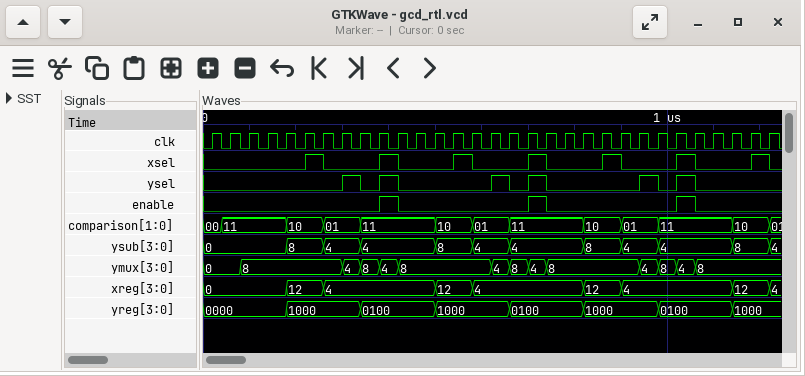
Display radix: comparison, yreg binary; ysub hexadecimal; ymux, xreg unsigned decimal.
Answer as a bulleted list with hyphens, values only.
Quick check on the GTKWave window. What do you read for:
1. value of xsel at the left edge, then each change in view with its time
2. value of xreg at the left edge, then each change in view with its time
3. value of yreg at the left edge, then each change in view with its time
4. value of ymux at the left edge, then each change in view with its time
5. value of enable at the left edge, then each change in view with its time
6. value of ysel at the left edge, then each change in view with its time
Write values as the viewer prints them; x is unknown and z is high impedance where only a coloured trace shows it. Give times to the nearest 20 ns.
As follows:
- 0, 1 at 220 ns, 0 at 260 ns, 1 at 380 ns, 0 at 420 ns, 1 at 540 ns, 0 at 580 ns, 1 at 700 ns, 0 at 740 ns, 1 at 860 ns, 0 at 900 ns, 1 at 1020 ns, 0 at 1060 ns, 1 at 1180 ns, 0 at 1220 ns
- 0, 12 at 180 ns, 4 at 260 ns, 12 at 500 ns, 4 at 580 ns, 12 at 820 ns, 4 at 900 ns, 12 at 1140 ns, 4 at 1220 ns
- 0000, 1000 at 180 ns, 0100 at 340 ns, 1000 at 500 ns, 0100 at 660 ns, 1000 at 820 ns, 0100 at 980 ns, 1000 at 1140 ns
- 0, 8 at 80 ns, 4 at 300 ns, 8 at 340 ns, 4 at 380 ns, 8 at 420 ns, 4 at 620 ns, 8 at 660 ns, 4 at 700 ns, 8 at 740 ns, 4 at 940 ns, 8 at 980 ns, 4 at 1020 ns, 8 at 1060 ns
- 0, 1 at 380 ns, 0 at 420 ns, 1 at 700 ns, 0 at 740 ns, 1 at 1020 ns, 0 at 1060 ns
- 0, 1 at 300 ns, 0 at 340 ns, 1 at 380 ns, 0 at 420 ns, 1 at 620 ns, 0 at 660 ns, 1 at 700 ns, 0 at 740 ns, 1 at 940 ns, 0 at 980 ns, 1 at 1020 ns, 0 at 1060 ns
